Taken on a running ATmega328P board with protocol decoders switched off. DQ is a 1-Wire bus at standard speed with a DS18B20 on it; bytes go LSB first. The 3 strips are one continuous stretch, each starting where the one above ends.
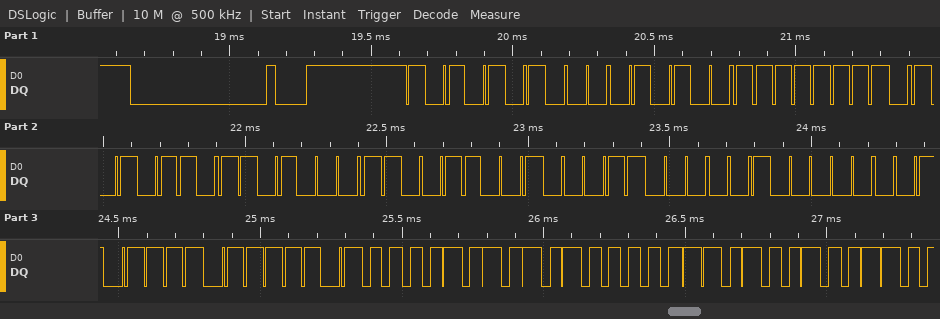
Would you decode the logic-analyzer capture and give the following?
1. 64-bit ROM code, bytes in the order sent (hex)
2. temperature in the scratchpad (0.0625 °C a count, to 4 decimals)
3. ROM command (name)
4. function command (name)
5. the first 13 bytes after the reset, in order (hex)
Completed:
28 FF 6A 8B 99 18 04 F4
85.0000 °C
Match ROM
Read Scratchpad
55 28 FF 6A 8B 99 18 04 F4 BE 50 05 4B
